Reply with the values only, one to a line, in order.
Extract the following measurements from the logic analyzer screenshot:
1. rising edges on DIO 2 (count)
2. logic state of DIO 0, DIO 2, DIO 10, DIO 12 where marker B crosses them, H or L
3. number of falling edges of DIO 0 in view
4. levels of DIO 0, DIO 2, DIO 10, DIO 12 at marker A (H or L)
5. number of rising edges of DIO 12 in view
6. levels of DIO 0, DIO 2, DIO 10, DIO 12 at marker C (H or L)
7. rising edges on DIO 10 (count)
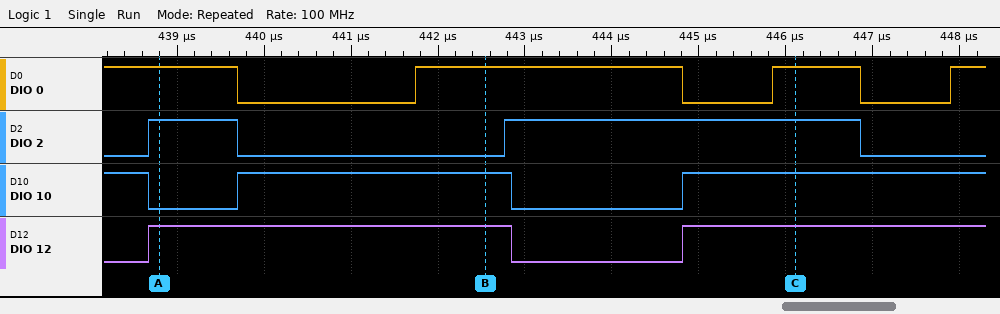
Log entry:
2
DIO 0=H, DIO 2=L, DIO 10=H, DIO 12=H
3
DIO 0=H, DIO 2=H, DIO 10=L, DIO 12=H
2
DIO 0=H, DIO 2=H, DIO 10=H, DIO 12=H
2
